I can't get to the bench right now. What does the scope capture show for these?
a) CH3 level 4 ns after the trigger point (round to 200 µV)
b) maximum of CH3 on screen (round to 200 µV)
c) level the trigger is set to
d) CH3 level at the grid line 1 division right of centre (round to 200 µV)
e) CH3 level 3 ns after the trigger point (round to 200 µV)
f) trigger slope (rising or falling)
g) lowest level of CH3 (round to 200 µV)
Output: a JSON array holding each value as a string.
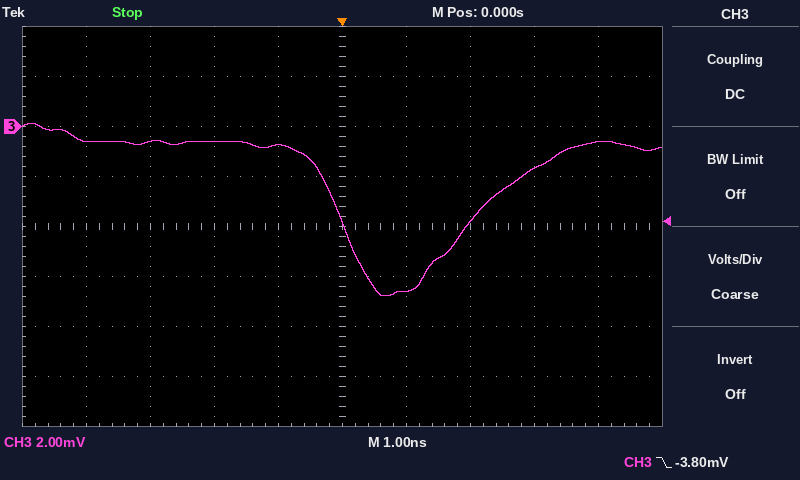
["-600 µV", "200 µV", "-3.80 mV", "-6.6 mV", "-1.6 mV", "falling", "-6.8 mV"]
